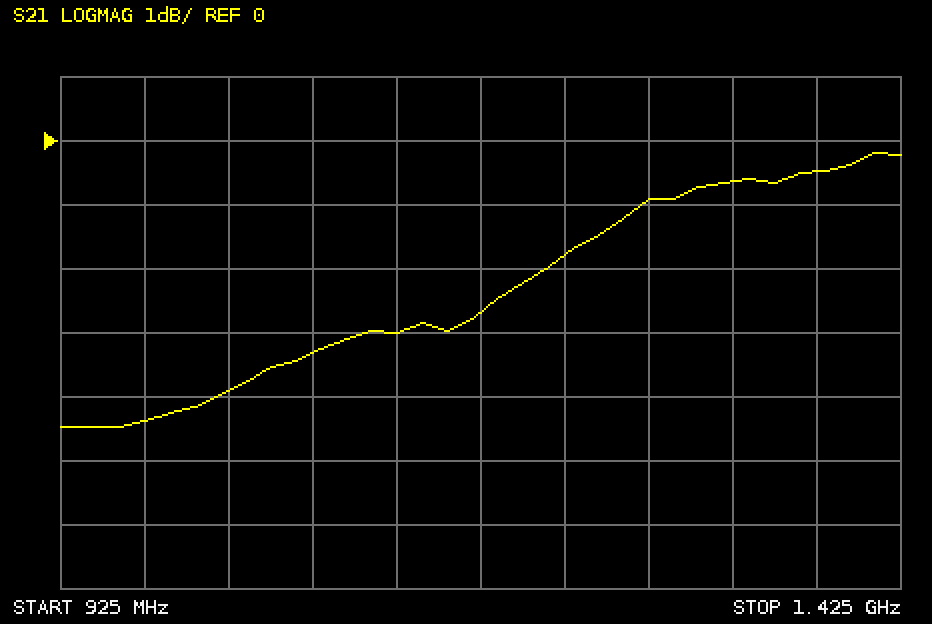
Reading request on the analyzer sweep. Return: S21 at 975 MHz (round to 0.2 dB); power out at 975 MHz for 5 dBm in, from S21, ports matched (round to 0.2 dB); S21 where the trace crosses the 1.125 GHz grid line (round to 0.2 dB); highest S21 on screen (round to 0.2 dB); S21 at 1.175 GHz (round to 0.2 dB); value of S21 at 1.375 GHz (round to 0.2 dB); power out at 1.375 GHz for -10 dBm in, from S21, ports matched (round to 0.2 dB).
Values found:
-4.4 dB
0.6 dBm
-3.0 dB
-0.2 dB
-2.6 dB
-0.4 dB
-10.4 dBm
